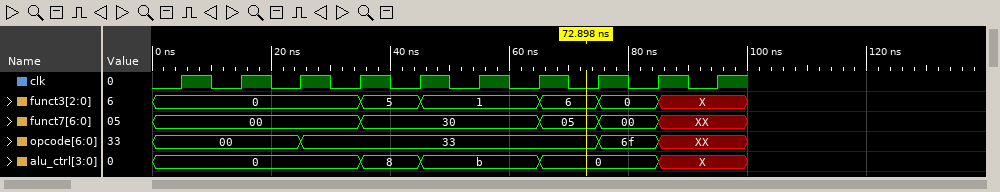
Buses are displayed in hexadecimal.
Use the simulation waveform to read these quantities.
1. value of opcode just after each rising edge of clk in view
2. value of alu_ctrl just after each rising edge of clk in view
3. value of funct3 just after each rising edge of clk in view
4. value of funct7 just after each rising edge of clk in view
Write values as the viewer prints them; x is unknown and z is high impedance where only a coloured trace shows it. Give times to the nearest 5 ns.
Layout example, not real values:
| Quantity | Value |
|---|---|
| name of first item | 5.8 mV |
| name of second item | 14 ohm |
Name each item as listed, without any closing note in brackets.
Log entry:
| Quantity | Value |
|---|---|
| value of opcode just after each rising edge of clk in view | 00, 00, 33, 33, 33, 33, 33, 6f, XX, XX |
| value of alu_ctrl just after each rising edge of clk in view | 0, 0, 0, 8, b, b, 0, 0, X, X |
| value of funct3 just after each rising edge of clk in view | 0, 0, 0, 5, 1, 1, 6, 0, X, X |
| value of funct7 just after each rising edge of clk in view | 00, 00, 00, 30, 30, 30, 05, 00, XX, XX |
